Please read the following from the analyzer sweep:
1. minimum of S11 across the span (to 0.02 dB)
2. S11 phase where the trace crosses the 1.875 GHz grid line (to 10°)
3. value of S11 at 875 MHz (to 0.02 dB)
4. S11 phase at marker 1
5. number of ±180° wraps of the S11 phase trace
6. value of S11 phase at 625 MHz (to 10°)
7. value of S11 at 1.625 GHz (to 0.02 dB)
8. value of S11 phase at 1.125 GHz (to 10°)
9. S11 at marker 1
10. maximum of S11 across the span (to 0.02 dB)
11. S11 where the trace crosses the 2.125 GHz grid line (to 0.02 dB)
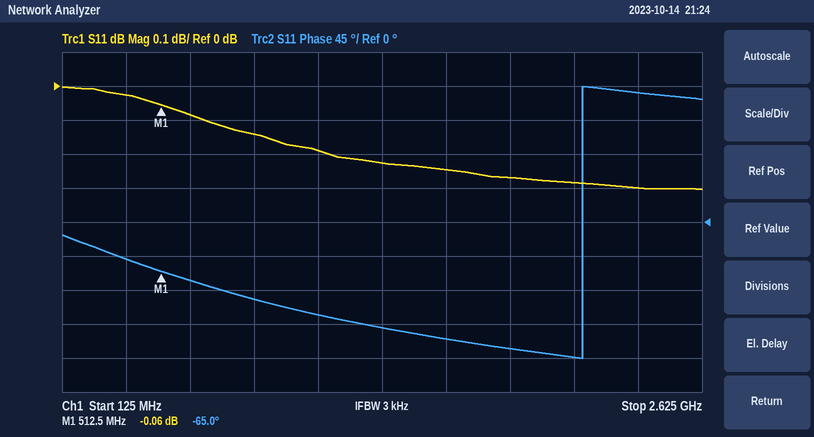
-0.30 dB
-170°
-0.14 dB
-65.0°
1
-80°
-0.24 dB
-120°
-0.06 dB
0.00 dB
-0.28 dB
